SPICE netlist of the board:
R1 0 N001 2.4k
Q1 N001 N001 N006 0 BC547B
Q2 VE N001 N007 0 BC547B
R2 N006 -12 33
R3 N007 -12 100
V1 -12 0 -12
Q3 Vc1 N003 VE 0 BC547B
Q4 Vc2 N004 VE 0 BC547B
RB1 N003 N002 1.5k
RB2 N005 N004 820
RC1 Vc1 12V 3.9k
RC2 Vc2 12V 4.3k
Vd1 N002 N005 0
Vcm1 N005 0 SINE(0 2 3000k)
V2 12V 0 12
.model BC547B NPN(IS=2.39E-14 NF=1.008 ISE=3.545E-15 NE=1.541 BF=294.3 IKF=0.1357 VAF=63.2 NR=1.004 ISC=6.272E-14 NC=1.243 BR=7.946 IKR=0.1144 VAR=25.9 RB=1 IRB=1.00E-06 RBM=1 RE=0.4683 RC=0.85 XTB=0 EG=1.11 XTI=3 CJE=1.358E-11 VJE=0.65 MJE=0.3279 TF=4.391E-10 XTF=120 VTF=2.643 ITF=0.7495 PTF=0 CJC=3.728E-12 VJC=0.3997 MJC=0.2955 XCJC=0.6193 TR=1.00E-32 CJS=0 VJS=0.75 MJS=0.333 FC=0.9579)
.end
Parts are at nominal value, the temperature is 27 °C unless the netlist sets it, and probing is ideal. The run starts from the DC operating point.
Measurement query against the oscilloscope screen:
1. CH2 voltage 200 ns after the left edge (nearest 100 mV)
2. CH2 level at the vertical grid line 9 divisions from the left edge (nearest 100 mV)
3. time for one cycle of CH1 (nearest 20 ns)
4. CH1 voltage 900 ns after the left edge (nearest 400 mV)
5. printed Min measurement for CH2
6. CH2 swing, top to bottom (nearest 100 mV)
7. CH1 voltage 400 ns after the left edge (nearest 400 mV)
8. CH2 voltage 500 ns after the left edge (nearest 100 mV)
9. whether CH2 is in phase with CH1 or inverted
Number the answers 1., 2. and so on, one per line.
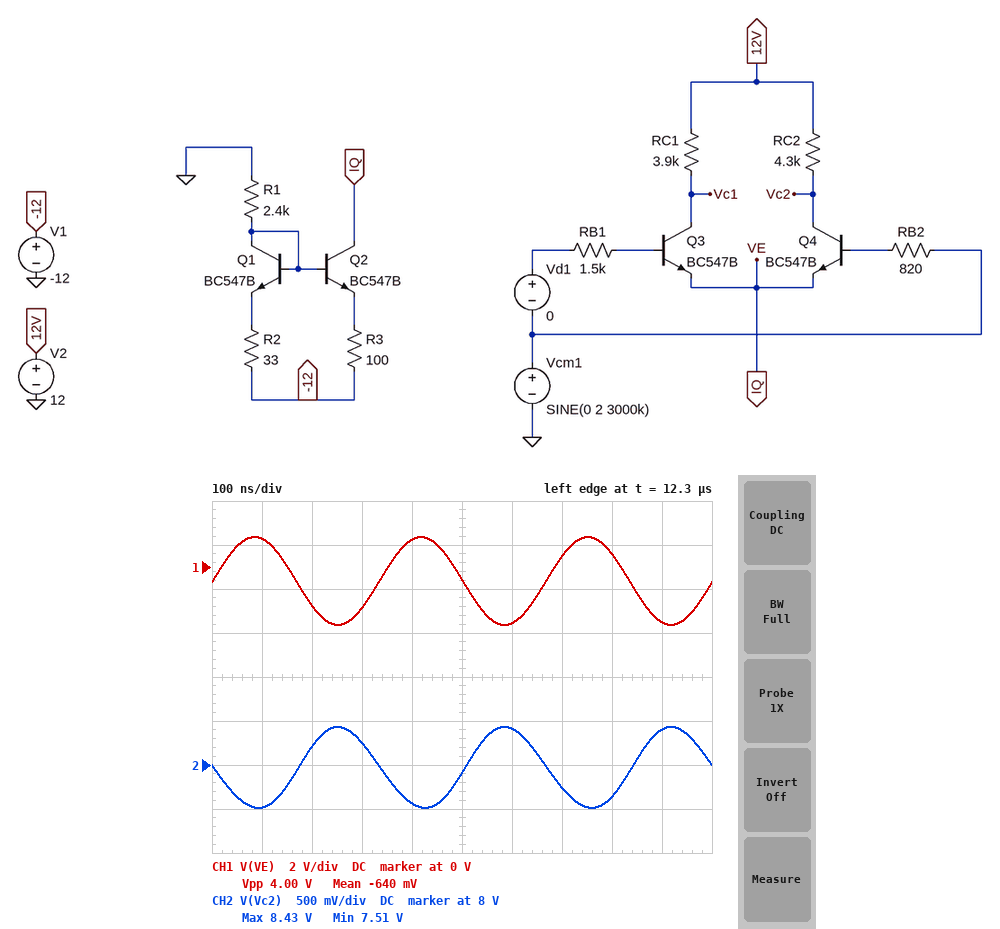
1. 8.2 V
2. 8.4 V
3. 340 ns
4. -2.4 V
5. 7.51 V
6. 900 mV
7. 1.2 V
8. 7.9 V
9. inverted
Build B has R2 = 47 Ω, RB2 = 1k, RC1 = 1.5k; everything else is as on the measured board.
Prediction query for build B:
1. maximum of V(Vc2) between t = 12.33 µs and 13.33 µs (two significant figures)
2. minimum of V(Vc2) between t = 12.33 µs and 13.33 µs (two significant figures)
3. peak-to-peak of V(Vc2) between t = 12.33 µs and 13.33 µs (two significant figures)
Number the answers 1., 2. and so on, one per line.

1. 7.2 V
2. 6.5 V
3. 650 mV
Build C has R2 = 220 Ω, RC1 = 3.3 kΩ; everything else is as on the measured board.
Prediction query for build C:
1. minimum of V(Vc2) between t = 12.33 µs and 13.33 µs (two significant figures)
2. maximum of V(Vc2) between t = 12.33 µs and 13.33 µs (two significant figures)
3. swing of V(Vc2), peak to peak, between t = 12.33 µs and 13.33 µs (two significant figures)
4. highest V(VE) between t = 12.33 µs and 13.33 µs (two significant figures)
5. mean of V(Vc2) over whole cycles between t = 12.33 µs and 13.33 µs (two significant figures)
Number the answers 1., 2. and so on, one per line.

1. -3.2 V
2. -140 mV
3. 3.1 V
4. -160 mV
5. -1.7 V
